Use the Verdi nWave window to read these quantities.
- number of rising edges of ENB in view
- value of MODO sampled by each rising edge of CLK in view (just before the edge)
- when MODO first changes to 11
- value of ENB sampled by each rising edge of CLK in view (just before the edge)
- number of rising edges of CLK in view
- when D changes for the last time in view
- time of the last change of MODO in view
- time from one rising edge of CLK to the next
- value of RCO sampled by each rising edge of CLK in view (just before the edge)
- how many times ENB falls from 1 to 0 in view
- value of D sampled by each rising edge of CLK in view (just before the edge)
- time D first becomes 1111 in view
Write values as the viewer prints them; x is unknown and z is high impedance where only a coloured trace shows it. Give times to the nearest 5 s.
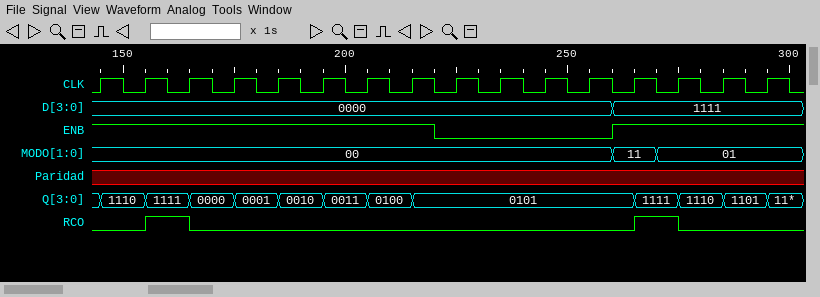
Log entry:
1
00, 00, 00, 00, 00, 00, 00, 00, 00, 00, 00, 00, 11, 01, 01, 01
260 s
1 1 1 1 1 1 1 1 0 0 0 0 1 1 1 1
16
260 s
270 s
10 s
0 0 1 0 0 0 0 0 0 0 0 0 0 1 0 0
1
0000, 0000, 0000, 0000, 0000, 0000, 0000, 0000, 0000, 0000, 0000, 0000, 1111, 1111, 1111, 1111
260 s
